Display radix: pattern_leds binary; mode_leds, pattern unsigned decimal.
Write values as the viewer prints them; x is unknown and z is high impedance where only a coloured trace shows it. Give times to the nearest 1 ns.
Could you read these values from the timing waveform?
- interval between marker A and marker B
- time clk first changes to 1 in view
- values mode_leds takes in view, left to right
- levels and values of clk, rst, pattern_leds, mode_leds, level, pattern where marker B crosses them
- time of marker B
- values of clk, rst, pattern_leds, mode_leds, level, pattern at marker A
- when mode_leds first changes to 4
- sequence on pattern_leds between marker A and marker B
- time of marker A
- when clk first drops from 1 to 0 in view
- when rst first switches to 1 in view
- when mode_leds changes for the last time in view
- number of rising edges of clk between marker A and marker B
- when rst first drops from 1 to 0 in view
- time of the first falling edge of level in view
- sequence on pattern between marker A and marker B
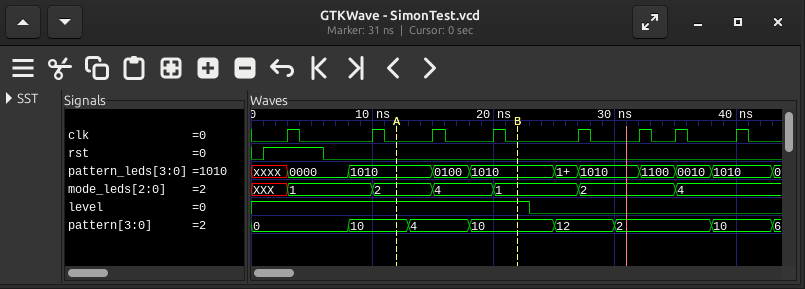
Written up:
10 ns
3 ns
XXX, 1, 2, 4, 1, 2, 4
clk=0, rst=0, pattern_leds=1010, mode_leds=1, level=1, pattern=10
22 ns
clk=0, rst=0, pattern_leds=1010, mode_leds=2, level=1, pattern=10
15 ns
1010, 0100, 1010
12 ns
4 ns
1 ns
35 ns
2
6 ns
23 ns
10, 4, 10
